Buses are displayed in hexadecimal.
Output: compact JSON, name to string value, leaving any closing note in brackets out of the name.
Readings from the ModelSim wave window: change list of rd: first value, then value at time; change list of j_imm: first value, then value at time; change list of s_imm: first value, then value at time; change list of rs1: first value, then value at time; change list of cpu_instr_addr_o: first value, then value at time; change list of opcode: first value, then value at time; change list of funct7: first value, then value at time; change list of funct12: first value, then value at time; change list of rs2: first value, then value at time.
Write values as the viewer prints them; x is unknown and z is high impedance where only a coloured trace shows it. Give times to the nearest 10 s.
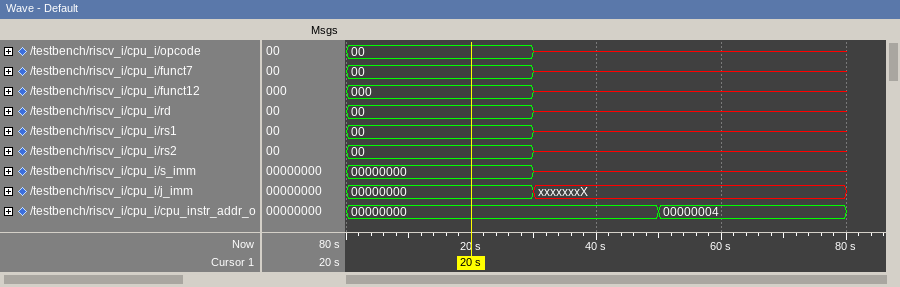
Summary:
{"change list of rd: first value, then value at time": "00, x at 30 s", "change list of j_imm: first value, then value at time": "00000000, xxxxxxxX at 30 s", "change list of s_imm: first value, then value at time": "00000000, x at 30 s", "change list of rs1: first value, then value at time": "00, x at 30 s", "change list of cpu_instr_addr_o: first value, then value at time": "00000000, 00000004 at 50 s", "change list of opcode: first value, then value at time": "00, x at 30 s", "change list of funct7: first value, then value at time": "00, x at 30 s", "change list of funct12: first value, then value at time": "000, x at 30 s", "change list of rs2: first value, then value at time": "00, x at 30 s"}
